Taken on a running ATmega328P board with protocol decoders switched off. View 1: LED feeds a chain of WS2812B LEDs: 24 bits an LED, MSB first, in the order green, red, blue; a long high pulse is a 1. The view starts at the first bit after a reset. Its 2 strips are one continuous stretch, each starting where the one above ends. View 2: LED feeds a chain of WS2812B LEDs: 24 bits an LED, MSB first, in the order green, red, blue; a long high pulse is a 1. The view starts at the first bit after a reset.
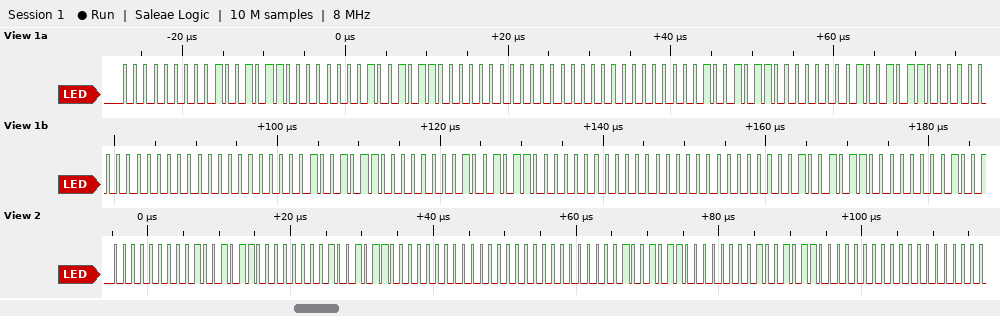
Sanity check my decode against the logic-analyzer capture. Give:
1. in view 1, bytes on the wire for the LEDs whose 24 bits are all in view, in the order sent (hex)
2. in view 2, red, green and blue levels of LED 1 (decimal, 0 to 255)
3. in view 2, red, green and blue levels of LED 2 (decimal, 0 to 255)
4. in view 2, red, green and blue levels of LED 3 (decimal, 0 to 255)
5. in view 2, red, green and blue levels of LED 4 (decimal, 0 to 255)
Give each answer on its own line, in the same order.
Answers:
00 4B 00 96 00 00 00 4B 00 96 00 00 00 4B 00 96 00 00 00 4B 00
75, 0, 0
0, 150, 0
75, 0, 0
0, 150, 0
